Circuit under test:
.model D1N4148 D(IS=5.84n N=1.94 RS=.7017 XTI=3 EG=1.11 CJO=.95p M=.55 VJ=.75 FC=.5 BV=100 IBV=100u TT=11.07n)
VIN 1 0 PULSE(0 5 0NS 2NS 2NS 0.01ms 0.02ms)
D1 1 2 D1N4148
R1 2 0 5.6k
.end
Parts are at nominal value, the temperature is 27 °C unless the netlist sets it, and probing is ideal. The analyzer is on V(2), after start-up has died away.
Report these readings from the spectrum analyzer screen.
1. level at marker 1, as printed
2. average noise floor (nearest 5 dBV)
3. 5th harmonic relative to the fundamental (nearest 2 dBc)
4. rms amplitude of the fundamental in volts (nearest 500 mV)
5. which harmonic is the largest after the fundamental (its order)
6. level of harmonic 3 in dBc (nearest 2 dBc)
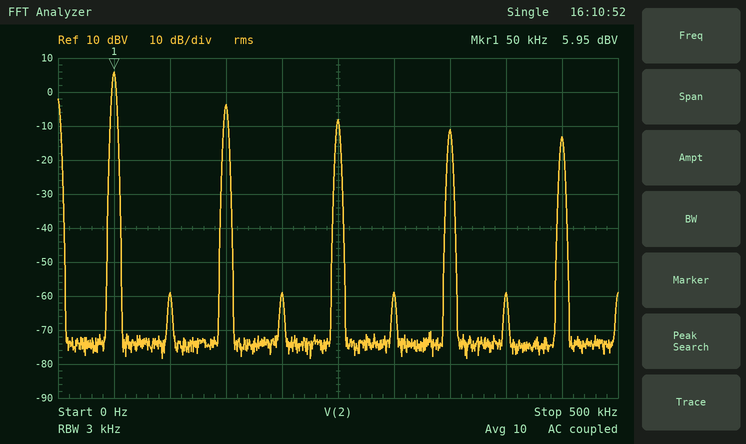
5.95 dBV
-75 dBV
-14 dBc
2.0 V
3
-10 dBc
